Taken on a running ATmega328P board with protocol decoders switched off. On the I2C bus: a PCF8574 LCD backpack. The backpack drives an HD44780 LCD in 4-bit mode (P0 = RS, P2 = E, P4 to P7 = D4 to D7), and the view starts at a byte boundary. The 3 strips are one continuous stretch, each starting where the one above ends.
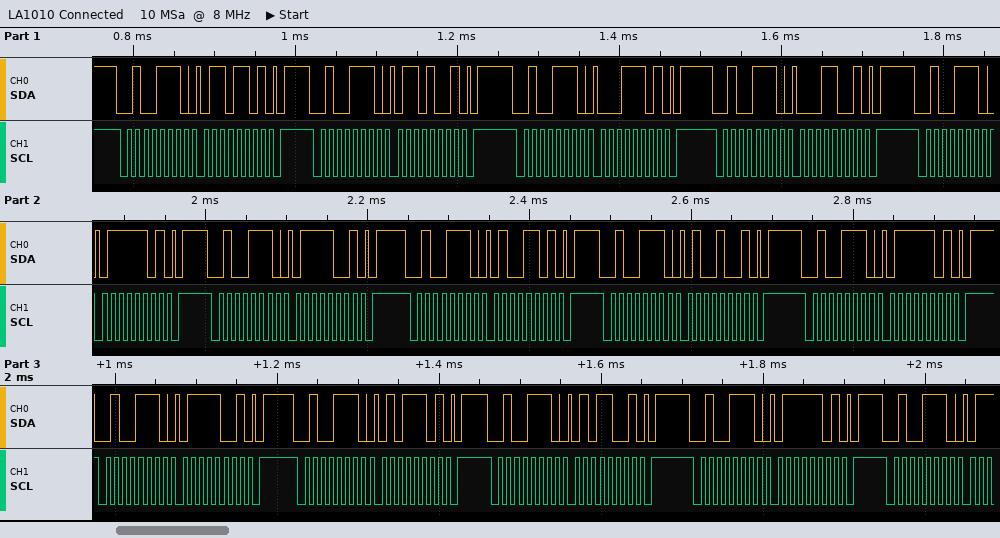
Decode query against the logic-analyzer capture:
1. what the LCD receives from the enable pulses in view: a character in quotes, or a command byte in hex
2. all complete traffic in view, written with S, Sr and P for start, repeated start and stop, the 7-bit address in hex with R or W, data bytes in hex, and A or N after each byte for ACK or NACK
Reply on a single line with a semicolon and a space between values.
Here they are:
'a' 't' 'u'; S 27W A 6D A P S 27W A 69 A P S 27W A 1D A P S 27W A 19 A P S 27W A 7D A P S 27W A 79 A P S 27W A 4D A P S 27W A 49 A P S 27W A 7D A P S 27W A 79 A P S 27W A 5D A P S 27W A 59 A P S 27W A 7D A P S 27W A
